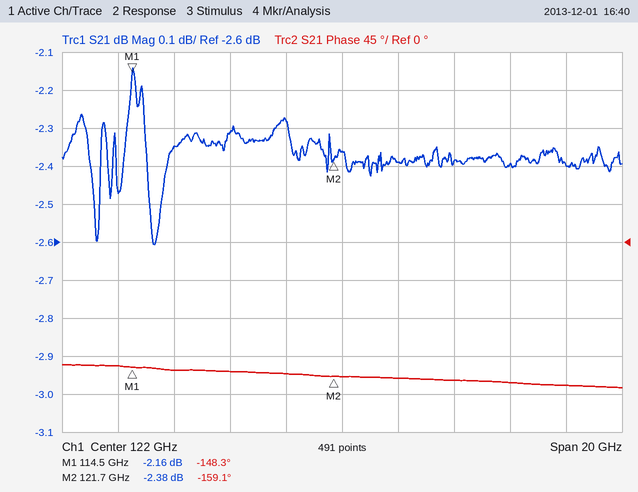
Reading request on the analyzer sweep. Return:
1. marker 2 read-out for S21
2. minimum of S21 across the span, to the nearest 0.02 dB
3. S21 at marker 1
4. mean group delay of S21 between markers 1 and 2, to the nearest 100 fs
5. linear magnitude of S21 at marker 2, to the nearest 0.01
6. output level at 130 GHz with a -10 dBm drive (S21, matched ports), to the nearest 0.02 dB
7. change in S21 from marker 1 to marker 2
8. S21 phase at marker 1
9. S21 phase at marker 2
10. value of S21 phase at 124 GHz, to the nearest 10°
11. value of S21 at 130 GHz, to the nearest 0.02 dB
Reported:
-2.38 dB
-2.60 dB
-2.16 dB
4.2 ps
0.76
-12.40 dBm
-0.22 dB
-148.3°
-159.1°
-160°
-2.40 dB
